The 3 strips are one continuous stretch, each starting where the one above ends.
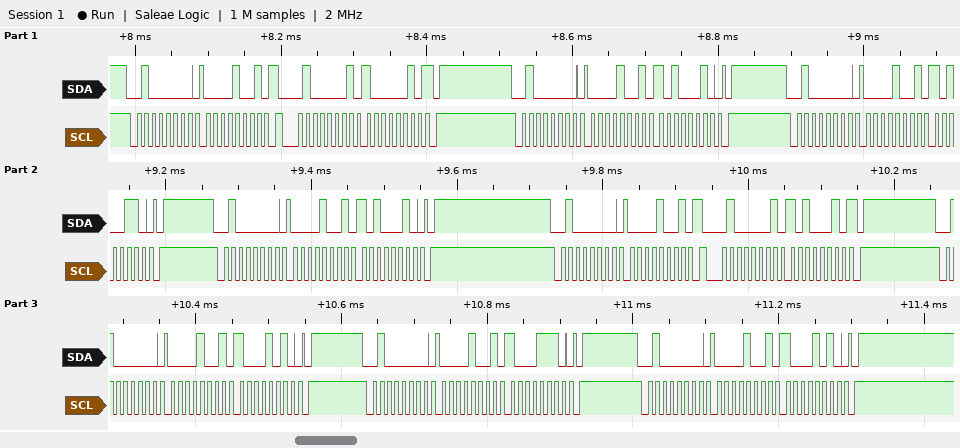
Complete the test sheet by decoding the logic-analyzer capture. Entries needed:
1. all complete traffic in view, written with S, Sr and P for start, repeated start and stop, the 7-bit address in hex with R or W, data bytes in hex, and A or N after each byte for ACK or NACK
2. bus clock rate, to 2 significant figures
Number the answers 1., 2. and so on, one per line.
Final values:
1. S 20W A 09 A Sr 20R A 82 N P S 20W A 09 A A2 A P S 20W A 09 A A6 A P S 20W A 09 A A2 A P S 20W A 09 A Sr 20R A A2 N P S 20W A 09 A 8A A P S 20W A 09 A 8E A P S 20W A 09 A 8A A P
2. 100 kHz
